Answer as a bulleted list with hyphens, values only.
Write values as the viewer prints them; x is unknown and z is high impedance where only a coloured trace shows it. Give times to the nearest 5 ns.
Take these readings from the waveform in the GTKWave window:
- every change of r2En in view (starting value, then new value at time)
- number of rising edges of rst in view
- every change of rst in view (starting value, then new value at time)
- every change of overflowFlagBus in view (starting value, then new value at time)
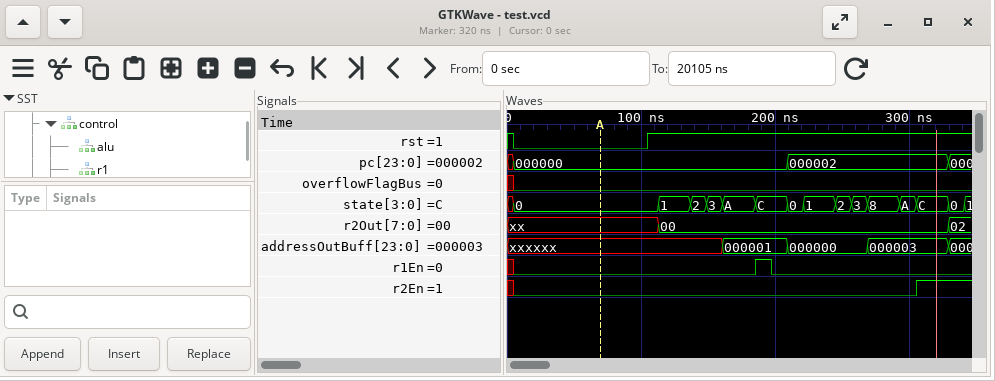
- x, 0 at 5 ns, 1 at 305 ns
- 1
- 1, 0 at 5 ns, 1 at 105 ns
- x, 0 at 5 ns
